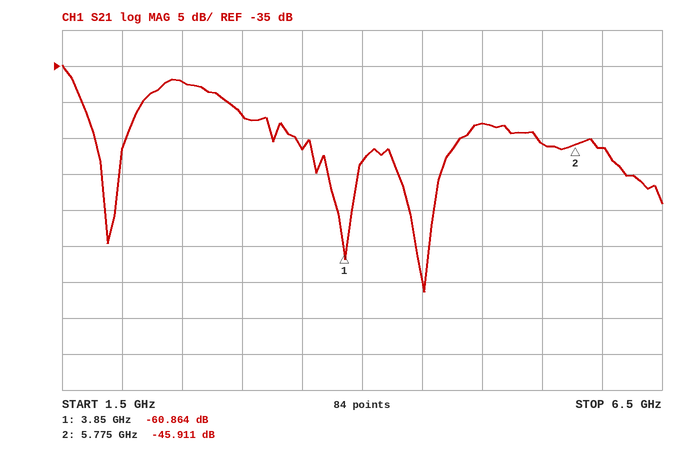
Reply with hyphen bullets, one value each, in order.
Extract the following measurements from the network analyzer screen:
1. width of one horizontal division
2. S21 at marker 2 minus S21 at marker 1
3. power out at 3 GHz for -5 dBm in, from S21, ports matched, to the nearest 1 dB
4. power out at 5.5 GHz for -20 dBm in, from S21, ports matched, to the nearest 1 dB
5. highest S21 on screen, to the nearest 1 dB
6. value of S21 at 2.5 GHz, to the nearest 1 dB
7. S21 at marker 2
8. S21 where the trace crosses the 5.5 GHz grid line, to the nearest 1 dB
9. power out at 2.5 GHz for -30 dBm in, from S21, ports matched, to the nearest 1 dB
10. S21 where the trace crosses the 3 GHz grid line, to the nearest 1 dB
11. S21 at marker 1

- 500 MHz
- 14.953 dB
- -47 dBm
- -66 dBm
- -35 dB
- -37 dB
- -45.911 dB
- -46 dB
- -67 dBm
- -42 dB
- -60.864 dB
